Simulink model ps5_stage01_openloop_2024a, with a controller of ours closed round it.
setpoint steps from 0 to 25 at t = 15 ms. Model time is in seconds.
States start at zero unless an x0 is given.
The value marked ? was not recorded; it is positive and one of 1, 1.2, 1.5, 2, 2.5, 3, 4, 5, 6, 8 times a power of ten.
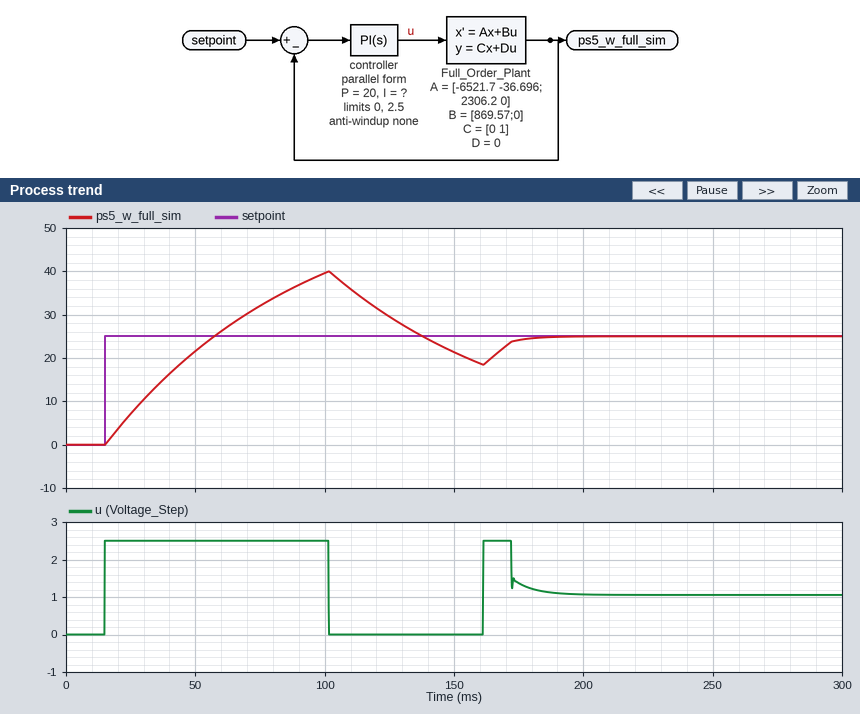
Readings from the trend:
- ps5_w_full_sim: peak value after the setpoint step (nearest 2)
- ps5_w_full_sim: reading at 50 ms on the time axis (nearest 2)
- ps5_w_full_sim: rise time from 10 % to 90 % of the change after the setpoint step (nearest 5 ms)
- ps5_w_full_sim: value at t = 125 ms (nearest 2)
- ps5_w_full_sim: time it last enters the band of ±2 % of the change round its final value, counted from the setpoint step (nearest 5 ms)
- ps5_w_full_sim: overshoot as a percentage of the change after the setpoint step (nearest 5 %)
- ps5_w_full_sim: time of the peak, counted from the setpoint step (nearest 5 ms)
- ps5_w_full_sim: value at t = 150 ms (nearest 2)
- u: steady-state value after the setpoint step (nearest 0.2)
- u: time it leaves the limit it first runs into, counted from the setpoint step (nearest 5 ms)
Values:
40
22
35 ms
30
165 ms
60 %
85 ms
22
1.0
85 ms
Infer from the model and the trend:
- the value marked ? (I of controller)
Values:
2500
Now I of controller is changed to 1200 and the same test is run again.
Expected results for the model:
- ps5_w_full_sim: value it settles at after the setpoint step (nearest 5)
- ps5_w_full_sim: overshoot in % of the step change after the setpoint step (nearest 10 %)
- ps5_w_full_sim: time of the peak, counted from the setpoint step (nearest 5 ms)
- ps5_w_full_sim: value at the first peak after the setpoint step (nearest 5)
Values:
25
50 %
80 ms
40
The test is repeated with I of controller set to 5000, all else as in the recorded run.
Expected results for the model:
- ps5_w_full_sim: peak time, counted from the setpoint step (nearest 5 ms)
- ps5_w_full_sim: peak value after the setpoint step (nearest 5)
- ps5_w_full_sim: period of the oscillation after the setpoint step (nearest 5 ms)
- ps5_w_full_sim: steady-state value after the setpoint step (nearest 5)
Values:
90 ms
40
105 ms
25
